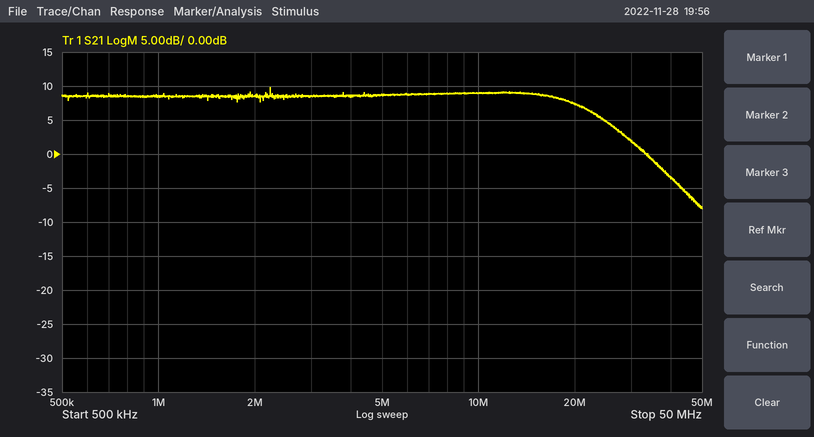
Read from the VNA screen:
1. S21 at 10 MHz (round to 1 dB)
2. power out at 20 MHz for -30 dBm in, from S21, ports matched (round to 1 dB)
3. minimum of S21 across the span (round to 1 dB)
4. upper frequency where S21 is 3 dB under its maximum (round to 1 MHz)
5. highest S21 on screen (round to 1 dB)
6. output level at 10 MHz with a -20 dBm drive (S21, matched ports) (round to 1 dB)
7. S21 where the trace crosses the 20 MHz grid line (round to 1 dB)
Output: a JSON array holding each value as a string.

["9 dB", "-23 dBm", "-8 dB", "21 MHz", "10 dB", "-11 dBm", "7 dB"]
